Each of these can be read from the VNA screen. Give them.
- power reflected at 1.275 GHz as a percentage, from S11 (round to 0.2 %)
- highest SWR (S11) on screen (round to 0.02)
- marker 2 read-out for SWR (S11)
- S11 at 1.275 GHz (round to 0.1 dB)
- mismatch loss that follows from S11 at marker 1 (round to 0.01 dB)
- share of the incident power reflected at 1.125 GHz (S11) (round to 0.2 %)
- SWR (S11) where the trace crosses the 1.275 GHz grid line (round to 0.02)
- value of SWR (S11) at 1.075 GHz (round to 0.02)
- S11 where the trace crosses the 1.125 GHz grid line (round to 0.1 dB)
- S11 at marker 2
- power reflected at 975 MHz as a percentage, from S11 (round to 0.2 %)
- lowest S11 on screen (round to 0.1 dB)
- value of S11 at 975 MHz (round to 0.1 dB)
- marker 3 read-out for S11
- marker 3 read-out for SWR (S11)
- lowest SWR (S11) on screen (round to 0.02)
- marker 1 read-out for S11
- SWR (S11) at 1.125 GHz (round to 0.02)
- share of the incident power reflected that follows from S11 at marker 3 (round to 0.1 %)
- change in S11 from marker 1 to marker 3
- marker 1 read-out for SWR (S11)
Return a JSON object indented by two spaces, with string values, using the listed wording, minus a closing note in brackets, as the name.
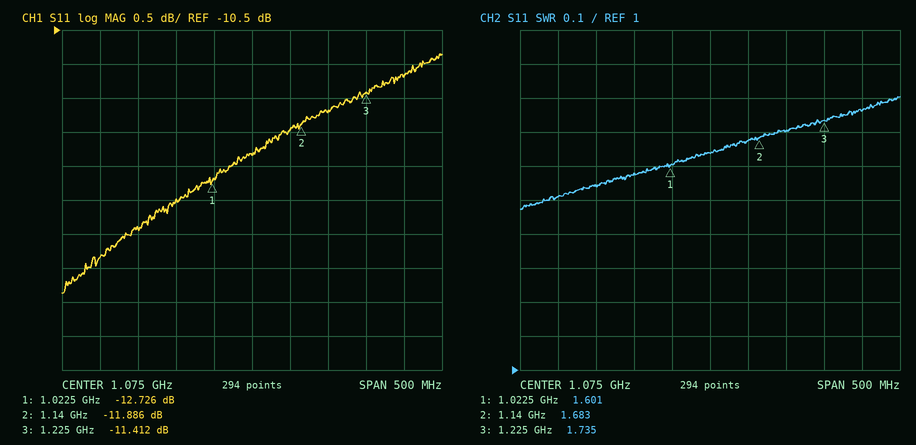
{
  "power reflected at 1.275 GHz as a percentage, from S11": "7.6 %",
  "highest SWR (S11) on screen": "1.80",
  "marker 2 read-out for SWR": "1.683",
  "S11 at 1.275 GHz": "-11.2 dB",
  "mismatch loss that follows from S11 at marker 1": "0.24 dB",
  "share of the incident power reflected at 1.125 GHz (S11)": "6.4 %",
  "SWR (S11) where the trace crosses the 1.275 GHz grid line": "1.76",
  "value of SWR (S11) at 1.075 GHz": "1.64",
  "S11 where the trace crosses the 1.125 GHz grid line": "-12.0 dB",
  "S11 at marker 2": "-11.886 dB",
  "power reflected at 975 MHz as a percentage, from S11": "5.0 %",
  "lowest S11 on screen": "-14.4 dB",
  "value of S11 at 975 MHz": "-13.0 dB",
  "marker 3 read-out for S11": "-11.412 dB",
  "marker 3 read-out for SWR": "1.735",
  "lowest SWR (S11) on screen": "1.48",
  "marker 1 read-out for S11": "-12.726 dB",
  "SWR (S11) at 1.125 GHz": "1.68",
  "share of the incident power reflected that follows from S11 at marker 3": "7.2 %",
  "change in S11 from marker 1 to marker 3": "1.314 dB",
  "marker 1 read-out for SWR": "1.601"
}
